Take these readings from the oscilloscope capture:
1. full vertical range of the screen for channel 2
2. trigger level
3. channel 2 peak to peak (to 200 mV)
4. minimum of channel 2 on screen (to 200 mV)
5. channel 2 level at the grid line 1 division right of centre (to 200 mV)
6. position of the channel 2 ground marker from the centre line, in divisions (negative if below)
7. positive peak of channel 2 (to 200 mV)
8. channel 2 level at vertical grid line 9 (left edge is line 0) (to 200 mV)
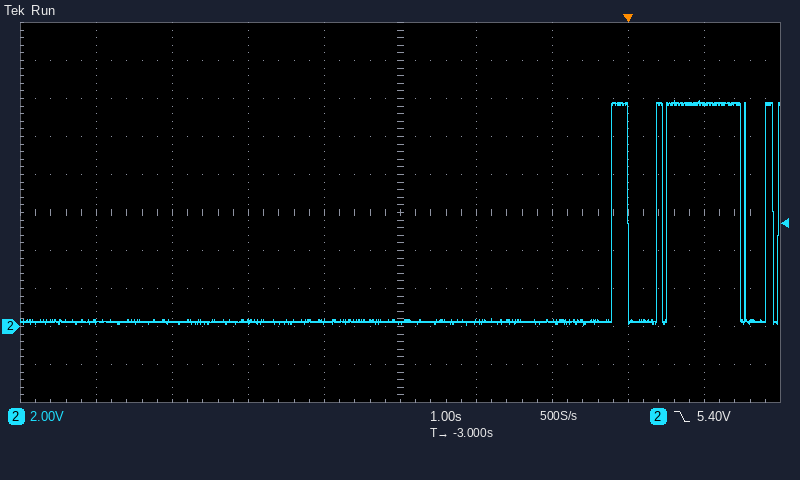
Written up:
20 V
5.40 V
11.8 V
0.0 V
200 mV
-3.0 div
11.8 V
11.8 V
